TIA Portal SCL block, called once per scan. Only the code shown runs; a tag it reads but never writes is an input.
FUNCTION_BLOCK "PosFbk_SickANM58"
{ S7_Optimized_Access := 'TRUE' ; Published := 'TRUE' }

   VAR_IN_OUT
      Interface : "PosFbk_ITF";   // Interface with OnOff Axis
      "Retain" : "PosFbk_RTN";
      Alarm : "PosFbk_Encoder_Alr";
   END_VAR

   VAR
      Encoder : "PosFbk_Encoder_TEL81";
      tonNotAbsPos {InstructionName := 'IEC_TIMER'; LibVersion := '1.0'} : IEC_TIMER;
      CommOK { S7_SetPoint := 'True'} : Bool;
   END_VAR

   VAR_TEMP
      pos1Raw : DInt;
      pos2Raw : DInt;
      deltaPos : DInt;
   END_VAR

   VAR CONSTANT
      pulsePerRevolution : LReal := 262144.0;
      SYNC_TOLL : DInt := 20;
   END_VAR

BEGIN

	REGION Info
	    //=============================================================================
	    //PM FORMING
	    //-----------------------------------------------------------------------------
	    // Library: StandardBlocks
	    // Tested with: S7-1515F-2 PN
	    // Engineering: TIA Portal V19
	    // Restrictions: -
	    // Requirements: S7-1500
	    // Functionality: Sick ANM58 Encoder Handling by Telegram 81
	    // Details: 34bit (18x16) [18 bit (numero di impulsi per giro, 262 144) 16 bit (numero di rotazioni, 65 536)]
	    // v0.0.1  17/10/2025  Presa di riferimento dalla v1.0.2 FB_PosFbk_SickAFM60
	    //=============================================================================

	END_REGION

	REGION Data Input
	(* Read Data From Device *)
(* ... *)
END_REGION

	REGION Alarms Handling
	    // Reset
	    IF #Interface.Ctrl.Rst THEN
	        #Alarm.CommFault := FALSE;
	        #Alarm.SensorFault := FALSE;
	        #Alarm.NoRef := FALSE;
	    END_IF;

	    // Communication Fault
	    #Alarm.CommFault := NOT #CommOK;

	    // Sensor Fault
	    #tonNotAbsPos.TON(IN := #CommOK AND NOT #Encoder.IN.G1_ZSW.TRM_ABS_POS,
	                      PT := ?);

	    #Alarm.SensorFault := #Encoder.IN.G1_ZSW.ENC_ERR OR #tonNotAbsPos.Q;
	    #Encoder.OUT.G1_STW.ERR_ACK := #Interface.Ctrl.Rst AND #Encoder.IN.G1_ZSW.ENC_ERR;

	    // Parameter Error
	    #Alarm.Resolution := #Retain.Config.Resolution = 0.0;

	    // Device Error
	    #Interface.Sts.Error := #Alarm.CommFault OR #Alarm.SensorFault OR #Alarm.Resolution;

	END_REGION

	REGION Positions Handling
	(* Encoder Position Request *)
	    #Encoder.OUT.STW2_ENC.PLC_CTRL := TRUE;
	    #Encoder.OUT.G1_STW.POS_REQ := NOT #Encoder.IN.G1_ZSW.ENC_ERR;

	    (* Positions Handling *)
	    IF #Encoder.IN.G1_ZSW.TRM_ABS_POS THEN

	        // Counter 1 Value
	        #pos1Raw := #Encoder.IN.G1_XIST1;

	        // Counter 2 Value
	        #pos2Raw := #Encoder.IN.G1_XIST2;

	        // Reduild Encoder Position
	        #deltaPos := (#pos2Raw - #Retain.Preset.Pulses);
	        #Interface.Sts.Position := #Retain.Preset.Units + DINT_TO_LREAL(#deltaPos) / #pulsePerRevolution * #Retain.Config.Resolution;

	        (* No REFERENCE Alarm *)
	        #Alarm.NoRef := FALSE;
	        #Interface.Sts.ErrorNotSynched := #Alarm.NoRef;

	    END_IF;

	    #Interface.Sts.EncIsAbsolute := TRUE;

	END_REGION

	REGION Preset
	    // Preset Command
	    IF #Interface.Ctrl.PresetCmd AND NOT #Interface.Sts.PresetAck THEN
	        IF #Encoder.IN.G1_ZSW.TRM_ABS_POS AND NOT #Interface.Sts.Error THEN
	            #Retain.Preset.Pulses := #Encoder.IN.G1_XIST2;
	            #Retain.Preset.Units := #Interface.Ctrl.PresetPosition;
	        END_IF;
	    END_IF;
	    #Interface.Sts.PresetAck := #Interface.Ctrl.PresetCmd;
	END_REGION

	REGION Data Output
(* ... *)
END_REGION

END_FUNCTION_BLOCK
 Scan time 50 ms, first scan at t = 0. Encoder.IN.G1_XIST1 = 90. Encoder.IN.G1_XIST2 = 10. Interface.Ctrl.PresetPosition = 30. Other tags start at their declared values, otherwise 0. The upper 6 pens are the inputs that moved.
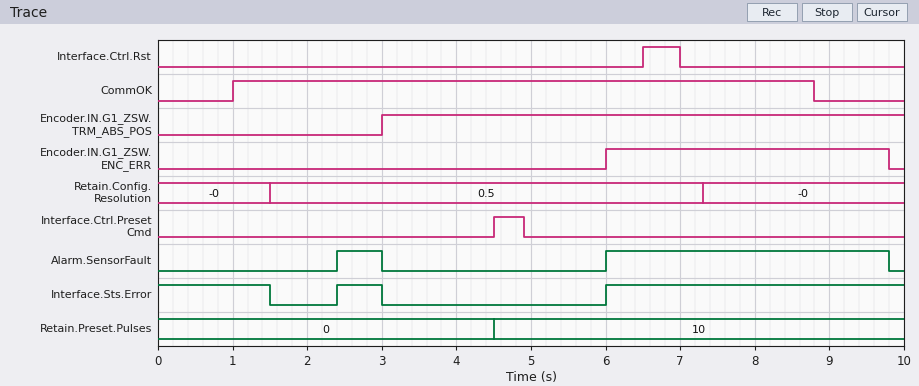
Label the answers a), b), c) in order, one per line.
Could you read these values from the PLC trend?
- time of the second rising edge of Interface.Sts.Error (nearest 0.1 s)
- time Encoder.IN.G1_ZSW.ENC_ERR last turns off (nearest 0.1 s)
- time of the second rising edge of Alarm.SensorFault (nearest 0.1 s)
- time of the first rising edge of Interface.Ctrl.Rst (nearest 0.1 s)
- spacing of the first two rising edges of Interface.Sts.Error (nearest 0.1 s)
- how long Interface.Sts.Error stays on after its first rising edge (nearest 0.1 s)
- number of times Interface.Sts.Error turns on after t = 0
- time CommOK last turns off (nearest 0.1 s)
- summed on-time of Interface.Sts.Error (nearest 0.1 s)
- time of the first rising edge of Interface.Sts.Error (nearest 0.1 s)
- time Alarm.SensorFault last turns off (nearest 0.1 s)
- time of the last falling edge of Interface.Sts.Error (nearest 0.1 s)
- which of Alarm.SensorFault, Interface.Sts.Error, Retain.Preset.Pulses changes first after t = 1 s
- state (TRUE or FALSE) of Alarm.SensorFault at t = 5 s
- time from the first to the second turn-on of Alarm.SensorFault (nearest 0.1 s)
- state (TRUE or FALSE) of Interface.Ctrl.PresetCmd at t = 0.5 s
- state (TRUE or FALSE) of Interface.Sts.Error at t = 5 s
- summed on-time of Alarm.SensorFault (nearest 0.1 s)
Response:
a) 6.0 s
b) 9.8 s
c) 6.0 s
d) 6.5 s
e) 3.6 s
f) 0.6 s
g) 2
h) 8.8 s
i) 6.1 s
j) 2.4 s
k) 9.8 s
l) 3.0 s
m) Interface.Sts.Error
n) FALSE
o) 3.6 s
p) FALSE
q) FALSE
r) 4.4 s
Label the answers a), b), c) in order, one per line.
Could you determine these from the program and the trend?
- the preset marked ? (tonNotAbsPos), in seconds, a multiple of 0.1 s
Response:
a) 1.4 s
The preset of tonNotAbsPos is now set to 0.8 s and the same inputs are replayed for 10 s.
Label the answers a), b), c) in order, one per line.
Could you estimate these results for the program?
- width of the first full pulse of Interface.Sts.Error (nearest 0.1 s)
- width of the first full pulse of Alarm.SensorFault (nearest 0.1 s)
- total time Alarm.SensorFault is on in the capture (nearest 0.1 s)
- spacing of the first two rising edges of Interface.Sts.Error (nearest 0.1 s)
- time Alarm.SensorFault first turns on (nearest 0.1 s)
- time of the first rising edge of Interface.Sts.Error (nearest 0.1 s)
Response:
a) 1.2 s
b) 1.2 s
c) 5.0 s
d) 4.2 s
e) 1.8 s
f) 1.8 s
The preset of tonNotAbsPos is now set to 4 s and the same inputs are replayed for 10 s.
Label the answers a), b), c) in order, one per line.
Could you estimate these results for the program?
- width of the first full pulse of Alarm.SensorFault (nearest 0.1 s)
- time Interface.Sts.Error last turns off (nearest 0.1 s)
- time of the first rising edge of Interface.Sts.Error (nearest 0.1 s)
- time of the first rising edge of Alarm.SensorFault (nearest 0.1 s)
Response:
a) 3.8 s
b) 1.5 s
c) 6.0 s
d) 6.0 s
